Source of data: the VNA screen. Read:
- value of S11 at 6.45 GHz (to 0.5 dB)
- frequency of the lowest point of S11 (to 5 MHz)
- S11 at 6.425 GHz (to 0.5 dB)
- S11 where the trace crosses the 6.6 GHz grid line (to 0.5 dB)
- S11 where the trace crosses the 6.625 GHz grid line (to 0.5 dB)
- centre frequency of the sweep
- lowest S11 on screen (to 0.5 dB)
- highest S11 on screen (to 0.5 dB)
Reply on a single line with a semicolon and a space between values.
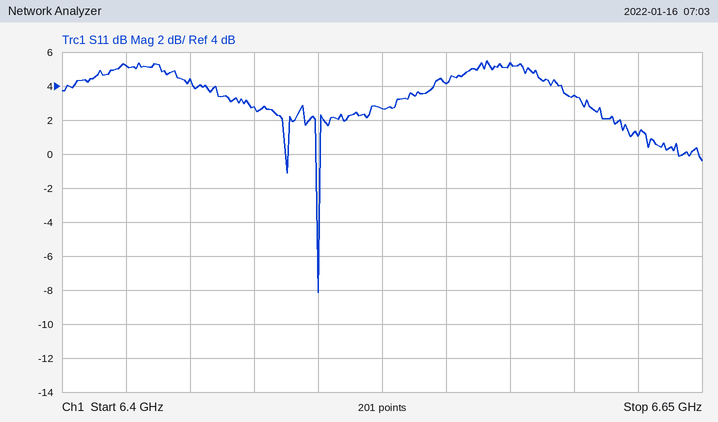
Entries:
4.5 dB; 6.500 GHz; 5.0 dB; 3.5 dB; 1.0 dB; 6.525 GHz; -8.0 dB; 5.5 dB
